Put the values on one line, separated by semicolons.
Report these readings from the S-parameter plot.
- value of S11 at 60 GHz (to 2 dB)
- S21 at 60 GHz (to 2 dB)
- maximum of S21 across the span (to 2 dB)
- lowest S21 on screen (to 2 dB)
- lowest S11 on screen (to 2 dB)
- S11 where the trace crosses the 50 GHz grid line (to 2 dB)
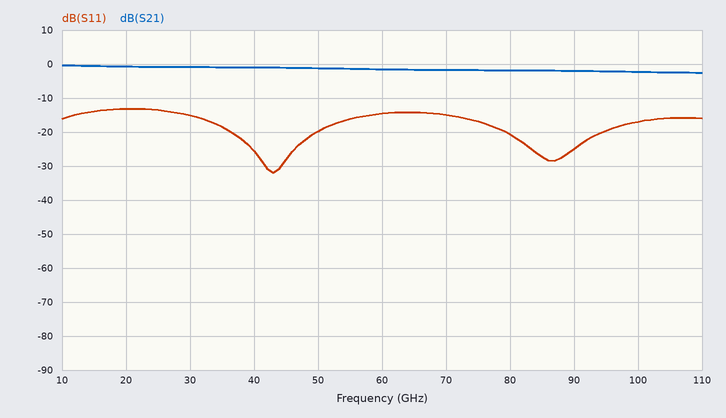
-14 dB; -2 dB; 0 dB; -2 dB; -32 dB; -20 dB
